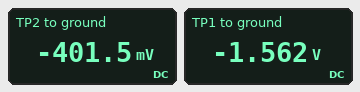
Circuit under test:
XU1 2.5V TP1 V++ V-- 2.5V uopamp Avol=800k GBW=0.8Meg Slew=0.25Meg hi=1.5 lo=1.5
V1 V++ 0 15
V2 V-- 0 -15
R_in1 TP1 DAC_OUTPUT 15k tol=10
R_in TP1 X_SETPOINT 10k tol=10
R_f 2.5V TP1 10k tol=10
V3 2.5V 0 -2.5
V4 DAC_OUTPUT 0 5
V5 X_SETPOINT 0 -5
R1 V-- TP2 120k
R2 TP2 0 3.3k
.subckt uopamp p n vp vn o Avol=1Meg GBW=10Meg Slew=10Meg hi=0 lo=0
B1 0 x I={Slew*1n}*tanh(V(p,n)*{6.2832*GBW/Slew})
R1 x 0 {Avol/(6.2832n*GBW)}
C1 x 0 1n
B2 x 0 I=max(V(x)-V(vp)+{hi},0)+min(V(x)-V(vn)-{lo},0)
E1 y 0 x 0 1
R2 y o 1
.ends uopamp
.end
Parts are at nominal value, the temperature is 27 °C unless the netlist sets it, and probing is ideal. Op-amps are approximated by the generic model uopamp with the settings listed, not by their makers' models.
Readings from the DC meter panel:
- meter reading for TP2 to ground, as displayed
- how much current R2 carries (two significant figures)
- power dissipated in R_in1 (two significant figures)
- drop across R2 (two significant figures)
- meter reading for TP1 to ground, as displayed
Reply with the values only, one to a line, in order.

-401.5 mV
120 µA
2.9 mW
400 mV
-1.562 V
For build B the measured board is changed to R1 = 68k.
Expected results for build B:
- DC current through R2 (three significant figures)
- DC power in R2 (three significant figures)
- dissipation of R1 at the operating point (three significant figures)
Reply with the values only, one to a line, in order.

210 µA
146 µW
3.01 mW
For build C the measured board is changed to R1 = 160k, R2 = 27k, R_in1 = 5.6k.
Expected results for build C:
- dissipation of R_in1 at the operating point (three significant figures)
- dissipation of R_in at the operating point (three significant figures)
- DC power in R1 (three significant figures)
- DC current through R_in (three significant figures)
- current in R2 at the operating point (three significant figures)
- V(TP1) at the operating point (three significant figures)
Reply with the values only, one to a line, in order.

3.82 mW
2.89 mW
1.03 mW
538 µA
80.2 µA
377 mV
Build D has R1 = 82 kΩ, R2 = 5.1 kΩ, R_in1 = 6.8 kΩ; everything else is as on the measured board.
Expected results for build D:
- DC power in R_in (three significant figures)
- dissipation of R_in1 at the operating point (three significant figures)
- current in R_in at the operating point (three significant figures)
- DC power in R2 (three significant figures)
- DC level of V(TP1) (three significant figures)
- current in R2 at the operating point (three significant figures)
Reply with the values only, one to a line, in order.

2.46 mW
3.74 mW
496 µA
151 µW
-42.4 mV
172 µA
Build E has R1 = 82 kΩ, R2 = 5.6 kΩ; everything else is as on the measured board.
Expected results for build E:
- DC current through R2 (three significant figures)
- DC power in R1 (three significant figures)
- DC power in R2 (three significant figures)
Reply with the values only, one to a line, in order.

171 µA
2.40 mW
164 µW
